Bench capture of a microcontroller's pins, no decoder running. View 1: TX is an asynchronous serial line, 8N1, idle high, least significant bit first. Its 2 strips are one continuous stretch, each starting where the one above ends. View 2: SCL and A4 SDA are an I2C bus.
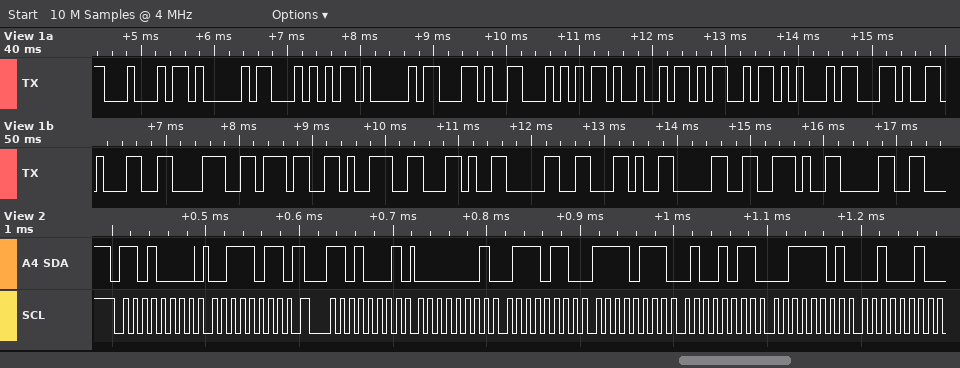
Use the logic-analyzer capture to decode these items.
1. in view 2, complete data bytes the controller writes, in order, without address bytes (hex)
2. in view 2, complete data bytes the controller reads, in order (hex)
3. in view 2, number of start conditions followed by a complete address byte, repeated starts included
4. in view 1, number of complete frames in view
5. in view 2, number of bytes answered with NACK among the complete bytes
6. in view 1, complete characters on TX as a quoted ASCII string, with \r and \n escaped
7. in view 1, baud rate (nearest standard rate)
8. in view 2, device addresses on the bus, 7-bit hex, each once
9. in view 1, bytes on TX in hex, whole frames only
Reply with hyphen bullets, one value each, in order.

- 3B
- 01 76 F7 4B 3D 22
- 2
- 20
- 0
- "DATA,TIME,1879,0,0.0"
- 9600 baud
- 0x68
- 44 41 54 41 2C 54 49 4D 45 2C 31 38 37 39 2C 30 2C 30 2E 30
